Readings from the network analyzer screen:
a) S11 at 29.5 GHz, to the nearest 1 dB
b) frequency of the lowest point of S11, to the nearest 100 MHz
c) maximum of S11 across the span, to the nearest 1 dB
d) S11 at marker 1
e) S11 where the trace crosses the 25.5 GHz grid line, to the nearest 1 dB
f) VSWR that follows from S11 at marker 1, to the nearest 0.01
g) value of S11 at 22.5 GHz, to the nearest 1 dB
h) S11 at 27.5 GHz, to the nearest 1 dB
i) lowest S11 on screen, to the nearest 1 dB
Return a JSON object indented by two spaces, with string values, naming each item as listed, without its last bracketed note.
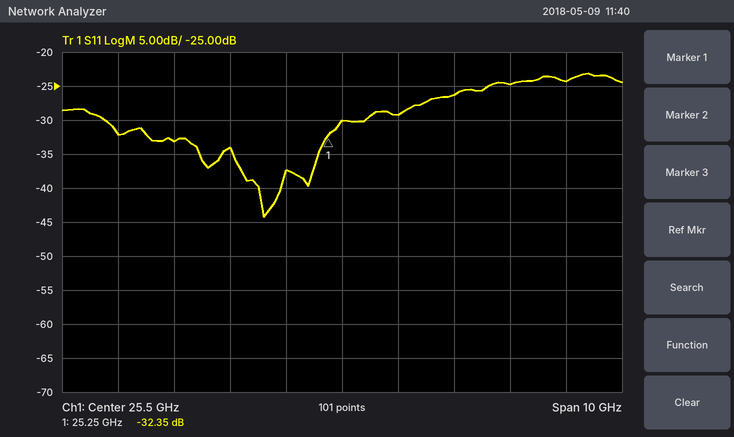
{
  "S11 at 29.5 GHz, to the nearest 1 dB": "-24 dB",
  "frequency of the lowest point of S11, to the nearest 100 MHz": "24.1 GHz",
  "maximum of S11 across the span, to the nearest 1 dB": "-23 dB",
  "S11 at marker 1": "-32.35 dB",
  "S11 where the trace crosses the 25.5 GHz grid line, to the nearest 1 dB": "-30 dB",
  "VSWR that follows from S11 at marker 1, to the nearest 0.01": "1.05",
  "value of S11 at 22.5 GHz, to the nearest 1 dB": "-33 dB",
  "S11 at 27.5 GHz, to the nearest 1 dB": "-26 dB",
  "lowest S11 on screen, to the nearest 1 dB": "-44 dB"
}
